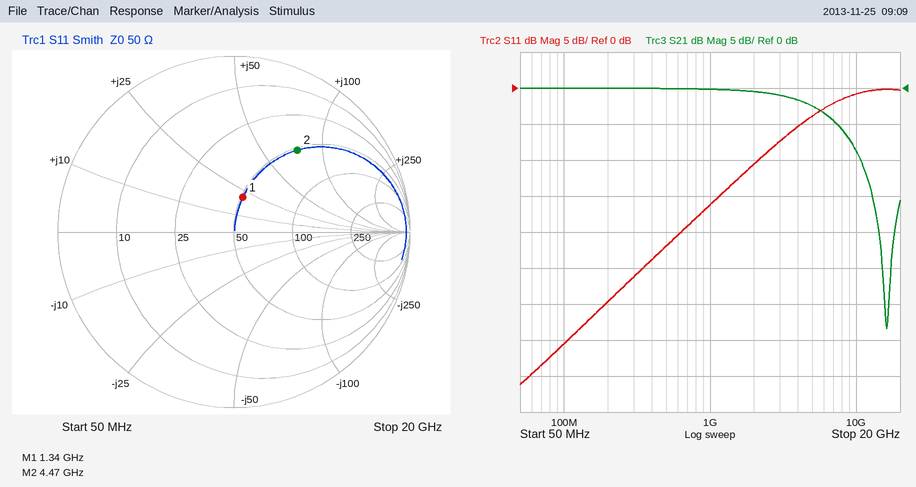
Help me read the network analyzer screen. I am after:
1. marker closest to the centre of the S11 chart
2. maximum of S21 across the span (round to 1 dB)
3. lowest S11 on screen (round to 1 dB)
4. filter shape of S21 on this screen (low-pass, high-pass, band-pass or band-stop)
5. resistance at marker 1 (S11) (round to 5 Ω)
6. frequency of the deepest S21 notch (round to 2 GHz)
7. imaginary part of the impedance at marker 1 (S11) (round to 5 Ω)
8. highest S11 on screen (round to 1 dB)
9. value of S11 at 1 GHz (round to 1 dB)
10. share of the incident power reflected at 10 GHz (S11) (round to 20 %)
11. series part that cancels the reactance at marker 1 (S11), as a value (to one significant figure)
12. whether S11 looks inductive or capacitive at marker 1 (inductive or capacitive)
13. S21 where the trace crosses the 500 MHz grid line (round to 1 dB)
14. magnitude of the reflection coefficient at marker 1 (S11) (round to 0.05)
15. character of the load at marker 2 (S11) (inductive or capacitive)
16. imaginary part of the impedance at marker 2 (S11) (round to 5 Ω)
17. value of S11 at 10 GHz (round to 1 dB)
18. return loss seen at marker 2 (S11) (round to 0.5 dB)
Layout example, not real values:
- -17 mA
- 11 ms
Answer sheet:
- marker 1
- 0 dB
- -41 dB
- low-pass
- 50 Ω
- 16 GHz
- +20 Ω
- 0 dB
- -16 dB
- 80 %
- 6 pF
- inductive
- 0 dB
- 0.20
- inductive
- +75 Ω
- -1 dB
- 4.5 dB
